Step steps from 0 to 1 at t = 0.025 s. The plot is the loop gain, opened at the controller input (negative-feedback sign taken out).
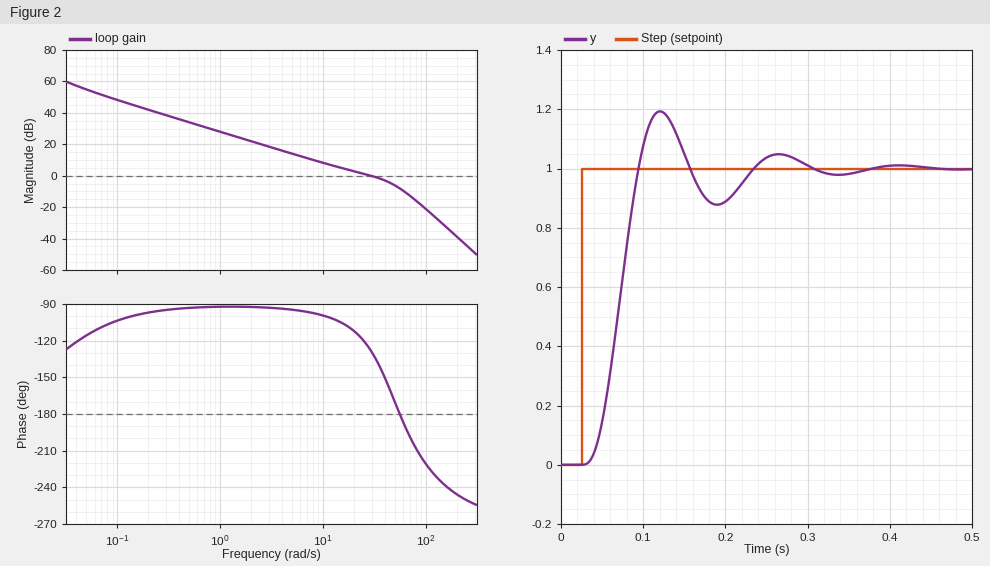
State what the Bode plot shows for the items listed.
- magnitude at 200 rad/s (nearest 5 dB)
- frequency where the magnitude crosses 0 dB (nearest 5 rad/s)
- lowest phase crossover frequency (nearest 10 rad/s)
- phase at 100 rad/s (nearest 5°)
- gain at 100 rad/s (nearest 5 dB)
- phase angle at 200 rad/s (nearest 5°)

-40 dB
30 rad/s
60 rad/s
-220°
-20 dB
-245°
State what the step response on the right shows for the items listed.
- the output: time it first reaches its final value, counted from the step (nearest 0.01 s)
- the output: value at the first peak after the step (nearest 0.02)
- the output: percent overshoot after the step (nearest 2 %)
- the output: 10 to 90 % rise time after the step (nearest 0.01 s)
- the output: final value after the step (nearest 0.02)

0.07 s
1.20
20 %
0.04 s
1.00
